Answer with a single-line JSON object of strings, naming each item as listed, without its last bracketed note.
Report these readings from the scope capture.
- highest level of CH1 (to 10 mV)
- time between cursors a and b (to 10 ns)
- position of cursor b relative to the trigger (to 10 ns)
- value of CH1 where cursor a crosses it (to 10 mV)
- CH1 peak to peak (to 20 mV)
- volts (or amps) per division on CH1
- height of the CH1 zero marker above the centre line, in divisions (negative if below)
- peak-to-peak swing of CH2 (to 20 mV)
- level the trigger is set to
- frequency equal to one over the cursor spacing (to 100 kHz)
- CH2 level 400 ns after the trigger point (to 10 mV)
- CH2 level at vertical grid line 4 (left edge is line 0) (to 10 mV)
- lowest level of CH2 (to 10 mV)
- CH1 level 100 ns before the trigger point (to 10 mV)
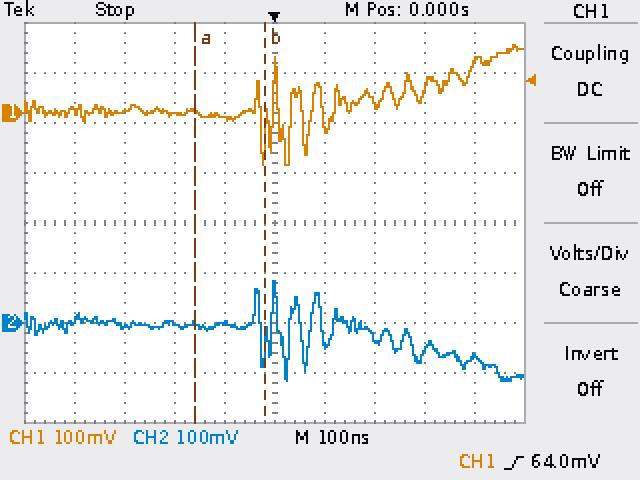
{"highest level of CH1": "140 mV", "time between cursors a and b": "140 ns", "position of cursor b relative to the trigger": "-20 ns", "value of CH1 where cursor a crosses it": "0 mV", "CH1 peak to peak": "240 mV", "volts (or amps) per division on CH1": "100 mV", "height of the CH1 zero marker above the centre line, in divisions": "+2.2 div", "peak-to-peak swing of CH2": "200 mV", "level the trigger is set to": "64.0 mV", "frequency equal to one over the cursor spacing": "7.1 MHz", "CH2 level 400 ns after the trigger point": "-70 mV", "CH2 level at vertical grid line 4 (left edge is line 0)": "0 mV", "lowest level of CH2": "-120 mV", "CH1 level 100 ns before the trigger point": "-10 mV"}
